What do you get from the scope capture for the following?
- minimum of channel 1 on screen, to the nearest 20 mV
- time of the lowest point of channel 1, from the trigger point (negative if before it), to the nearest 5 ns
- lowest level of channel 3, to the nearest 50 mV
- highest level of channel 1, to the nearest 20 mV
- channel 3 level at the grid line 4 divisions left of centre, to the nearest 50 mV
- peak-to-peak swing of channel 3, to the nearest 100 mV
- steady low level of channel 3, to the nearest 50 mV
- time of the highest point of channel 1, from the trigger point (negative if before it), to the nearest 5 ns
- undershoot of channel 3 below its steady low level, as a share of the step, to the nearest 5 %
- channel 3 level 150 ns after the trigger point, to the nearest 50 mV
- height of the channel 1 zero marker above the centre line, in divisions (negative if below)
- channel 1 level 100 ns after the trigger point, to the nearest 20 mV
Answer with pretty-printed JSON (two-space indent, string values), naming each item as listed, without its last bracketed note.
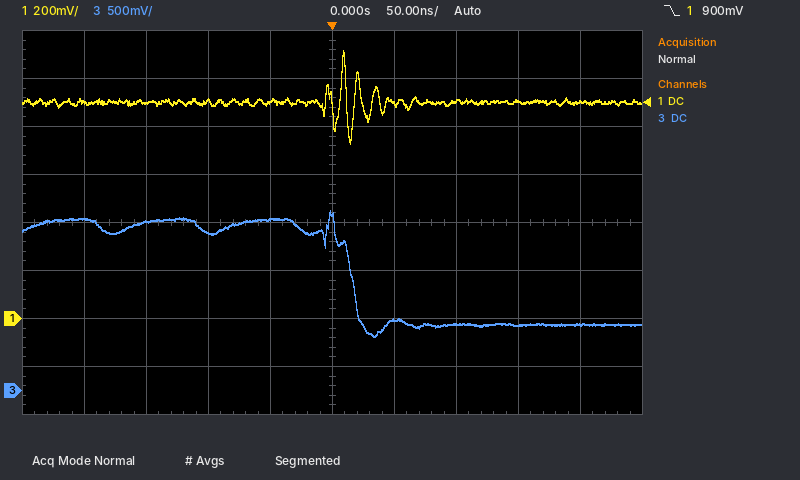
{
  "minimum of channel 1 on screen, to the nearest 20 mV": "720 mV",
  "time of the lowest point of channel 1, from the trigger point (negative if before it), to the nearest 5 ns": "+15 ns",
  "lowest level of channel 3, to the nearest 50 mV": "550 mV",
  "highest level of channel 1, to the nearest 20 mV": "1.12 V",
  "channel 3 level at the grid line 4 divisions left of centre, to the nearest 50 mV": "1.80 V",
  "peak-to-peak swing of channel 3, to the nearest 100 mV": "1.30 V",
  "steady low level of channel 3, to the nearest 50 mV": "700 mV",
  "time of the highest point of channel 1, from the trigger point (negative if before it), to the nearest 5 ns": "+10 ns",
  "undershoot of channel 3 below its steady low level, as a share of the step, to the nearest 5 %": "10 %",
  "channel 3 level 150 ns after the trigger point, to the nearest 50 mV": "700 mV",
  "height of the channel 1 zero marker above the centre line, in divisions": "-2.0 div",
  "channel 1 level 100 ns after the trigger point, to the nearest 20 mV": "900 mV"
}
